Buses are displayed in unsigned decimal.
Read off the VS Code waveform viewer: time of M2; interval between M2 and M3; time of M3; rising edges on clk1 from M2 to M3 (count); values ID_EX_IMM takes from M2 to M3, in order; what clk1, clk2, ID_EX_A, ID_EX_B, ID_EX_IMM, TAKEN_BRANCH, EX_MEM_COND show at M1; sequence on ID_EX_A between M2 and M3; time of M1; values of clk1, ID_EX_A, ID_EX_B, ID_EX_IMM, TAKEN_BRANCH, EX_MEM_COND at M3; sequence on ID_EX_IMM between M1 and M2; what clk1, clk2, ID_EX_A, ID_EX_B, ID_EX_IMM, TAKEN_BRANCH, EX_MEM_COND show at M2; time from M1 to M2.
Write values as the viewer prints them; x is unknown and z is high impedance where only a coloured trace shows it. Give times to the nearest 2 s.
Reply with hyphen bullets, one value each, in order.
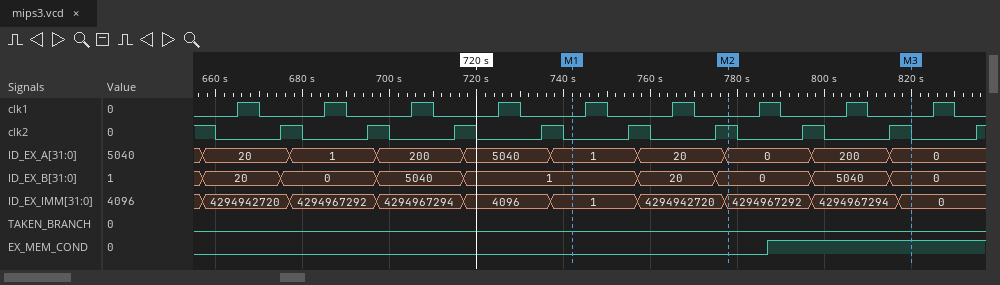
- 778 s
- 42 s
- 820 s
- 2
- 4294967292, 4294967294, 0
- clk1=0, clk2=0, ID_EX_A=1, ID_EX_B=1, ID_EX_IMM=1, TAKEN_BRANCH=0, EX_MEM_COND=0
- 0, 200, 0
- 742 s
- clk1=0, ID_EX_A=0, ID_EX_B=0, ID_EX_IMM=0, TAKEN_BRANCH=0, EX_MEM_COND=1
- 1, 4294942720, 4294967292
- clk1=0, clk2=1, ID_EX_A=0, ID_EX_B=0, ID_EX_IMM=4294967292, TAKEN_BRANCH=0, EX_MEM_COND=0
- 36 s
